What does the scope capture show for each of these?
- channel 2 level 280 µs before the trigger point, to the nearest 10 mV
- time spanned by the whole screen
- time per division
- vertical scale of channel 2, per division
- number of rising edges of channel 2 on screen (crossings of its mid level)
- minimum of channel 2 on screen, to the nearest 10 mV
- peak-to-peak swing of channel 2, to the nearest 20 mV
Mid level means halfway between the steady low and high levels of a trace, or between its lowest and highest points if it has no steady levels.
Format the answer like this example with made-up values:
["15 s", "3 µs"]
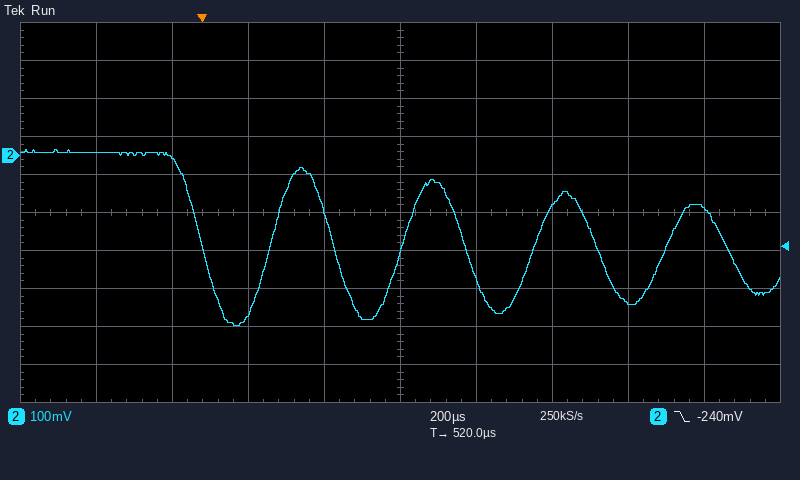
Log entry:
["10 mV", "2 ms", "200 µs", "100 mV", "4", "-450 mV", "460 mV"]
